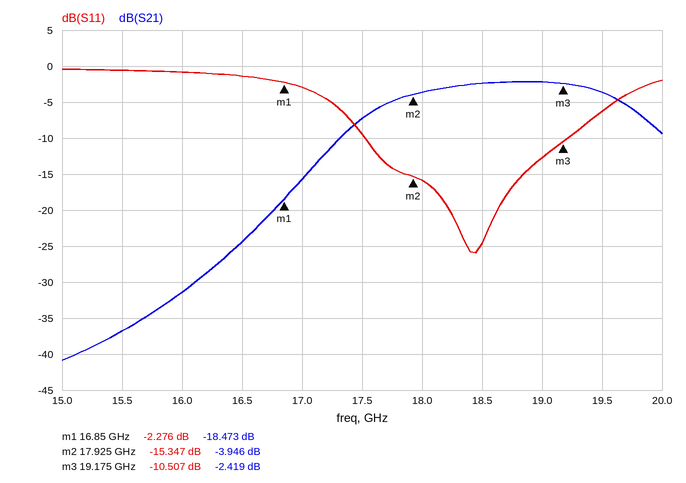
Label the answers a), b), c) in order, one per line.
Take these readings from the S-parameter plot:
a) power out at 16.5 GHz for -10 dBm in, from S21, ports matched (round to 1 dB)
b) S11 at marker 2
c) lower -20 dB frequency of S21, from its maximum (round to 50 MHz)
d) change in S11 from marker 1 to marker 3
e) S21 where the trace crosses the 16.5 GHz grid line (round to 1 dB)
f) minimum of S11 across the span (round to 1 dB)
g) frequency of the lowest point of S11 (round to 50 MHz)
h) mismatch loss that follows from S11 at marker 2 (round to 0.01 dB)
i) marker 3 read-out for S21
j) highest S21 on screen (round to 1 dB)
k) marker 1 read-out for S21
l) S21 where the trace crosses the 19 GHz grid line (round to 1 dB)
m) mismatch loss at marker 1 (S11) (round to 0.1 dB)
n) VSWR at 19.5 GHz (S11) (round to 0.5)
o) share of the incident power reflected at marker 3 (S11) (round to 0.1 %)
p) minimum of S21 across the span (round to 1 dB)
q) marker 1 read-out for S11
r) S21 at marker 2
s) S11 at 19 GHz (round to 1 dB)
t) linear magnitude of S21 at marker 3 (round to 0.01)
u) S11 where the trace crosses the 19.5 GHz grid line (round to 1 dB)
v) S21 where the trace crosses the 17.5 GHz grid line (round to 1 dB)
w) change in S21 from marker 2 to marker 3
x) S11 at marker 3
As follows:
a) -34 dBm
b) -15.347 dB
c) 16.65 GHz
d) -8.231 dB
e) -24 dB
f) -26 dB
g) 18.45 GHz
h) 0.13 dB
i) -2.419 dB
j) -2 dB
k) -18.473 dB
l) -2 dB
m) 3.9 dB
n) 3.0
o) 8.9 %
p) -41 dB
q) -2.276 dB
r) -3.946 dB
s) -13 dB
t) 0.76
u) -6 dB
v) -7 dB
w) 1.527 dB
x) -10.507 dB
